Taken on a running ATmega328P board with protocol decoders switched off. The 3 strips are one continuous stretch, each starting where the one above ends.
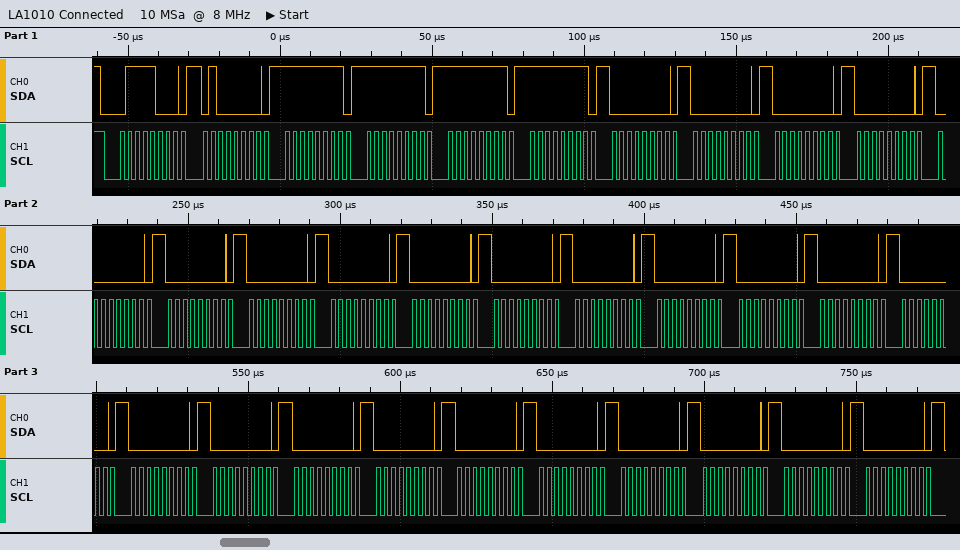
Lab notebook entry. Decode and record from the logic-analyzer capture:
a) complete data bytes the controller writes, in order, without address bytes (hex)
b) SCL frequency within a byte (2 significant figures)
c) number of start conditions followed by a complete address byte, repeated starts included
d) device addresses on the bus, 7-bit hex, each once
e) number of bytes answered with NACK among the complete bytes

40 FF FF FF FF 00 00 00 00 00 00 00 00 00 00 00 00 00 00 00 00 00 00 00 00 00 00 00 00 00
400 kHz
1
0x3C
0
